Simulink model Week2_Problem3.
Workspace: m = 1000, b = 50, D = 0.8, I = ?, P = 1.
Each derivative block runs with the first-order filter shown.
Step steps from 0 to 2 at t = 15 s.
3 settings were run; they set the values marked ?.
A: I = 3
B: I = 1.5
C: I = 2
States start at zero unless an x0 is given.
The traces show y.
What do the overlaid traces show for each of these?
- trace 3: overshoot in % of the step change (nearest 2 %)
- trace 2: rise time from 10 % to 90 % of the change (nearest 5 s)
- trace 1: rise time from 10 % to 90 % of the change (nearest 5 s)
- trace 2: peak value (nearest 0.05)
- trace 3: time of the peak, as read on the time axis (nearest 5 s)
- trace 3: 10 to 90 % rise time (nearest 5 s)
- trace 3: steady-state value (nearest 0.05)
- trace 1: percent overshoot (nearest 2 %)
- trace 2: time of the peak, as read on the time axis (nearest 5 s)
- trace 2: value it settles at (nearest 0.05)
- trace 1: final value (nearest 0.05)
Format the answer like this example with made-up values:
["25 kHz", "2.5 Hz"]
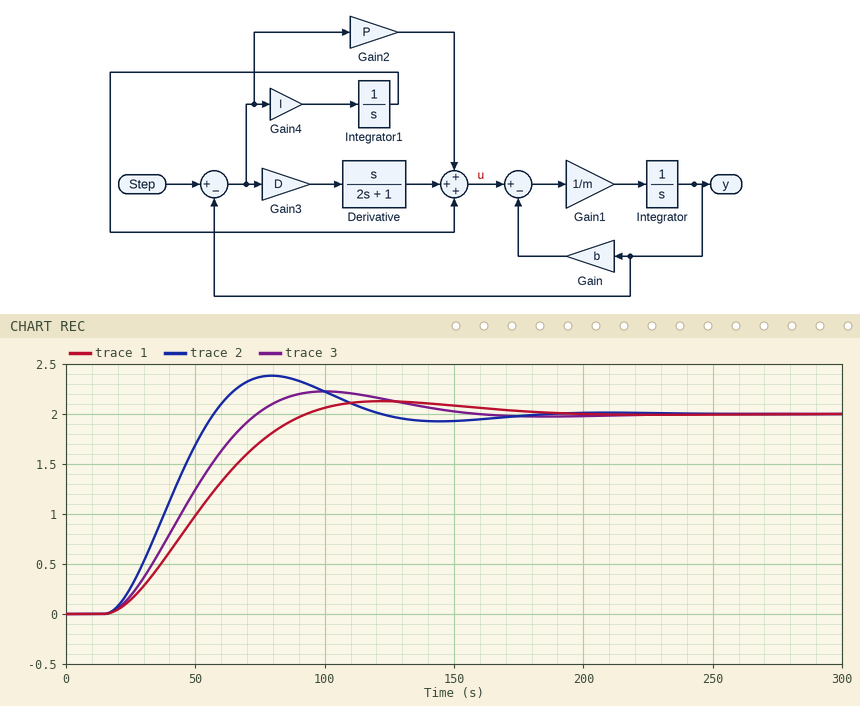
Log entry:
["12 %", "30 s", "50 s", "2.40", "100 s", "40 s", "2.00", "6 %", "80 s", "2.00", "2.00"]
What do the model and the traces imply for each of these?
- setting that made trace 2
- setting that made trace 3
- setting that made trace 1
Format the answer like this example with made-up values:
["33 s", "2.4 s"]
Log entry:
["A", "C", "B"]
